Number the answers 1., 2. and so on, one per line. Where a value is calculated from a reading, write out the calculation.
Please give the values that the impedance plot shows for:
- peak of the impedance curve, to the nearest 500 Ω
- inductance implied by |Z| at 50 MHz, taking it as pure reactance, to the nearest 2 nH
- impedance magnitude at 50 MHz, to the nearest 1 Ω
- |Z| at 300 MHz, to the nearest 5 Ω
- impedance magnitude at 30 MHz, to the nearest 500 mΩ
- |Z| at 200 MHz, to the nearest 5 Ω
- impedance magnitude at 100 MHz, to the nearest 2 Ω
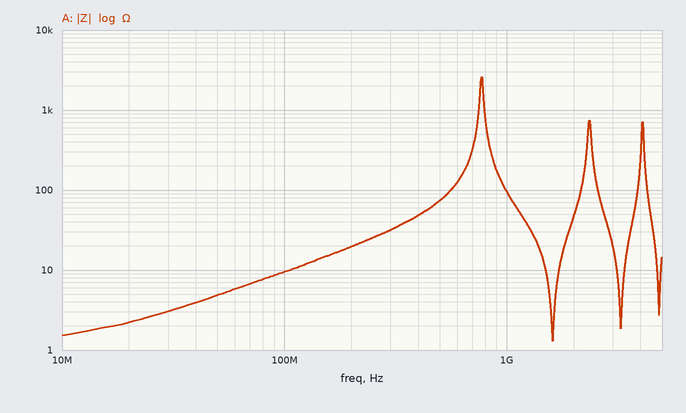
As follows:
1. 2.5 kΩ
2. L = 5 Ω/(2π × 50 MHz) ≈ 16 nH
3. 5 Ω
4. 30 Ω
5. 3.0 Ω
6. 20 Ω
7. 10 Ω
